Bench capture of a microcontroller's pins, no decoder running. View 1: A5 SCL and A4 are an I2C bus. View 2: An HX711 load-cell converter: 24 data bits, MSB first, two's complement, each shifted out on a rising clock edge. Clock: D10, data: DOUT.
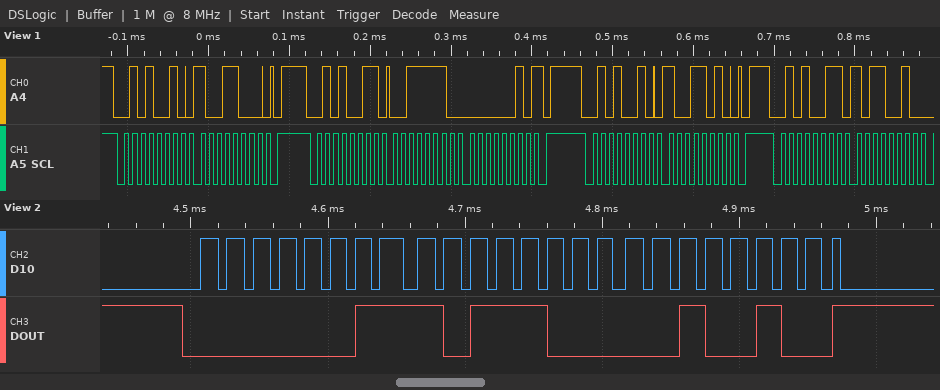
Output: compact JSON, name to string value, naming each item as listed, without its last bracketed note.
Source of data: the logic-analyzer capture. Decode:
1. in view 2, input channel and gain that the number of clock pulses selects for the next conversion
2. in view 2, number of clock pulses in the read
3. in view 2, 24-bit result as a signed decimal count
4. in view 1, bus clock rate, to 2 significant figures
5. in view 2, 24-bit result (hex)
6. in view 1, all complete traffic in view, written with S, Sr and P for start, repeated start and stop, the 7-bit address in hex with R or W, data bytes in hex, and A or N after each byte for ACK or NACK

{"in view 2, input channel and gain that the number of clock pulses selects for the next conversion": "channel A, gain 128", "in view 2, number of clock pulses in the read": "25", "in view 2, 24-bit result as a signed decimal count": "243748", "in view 1, bus clock rate, to 2 significant figures": "100 kHz", "in view 2, 24-bit result": "0x03B824", "in view 1, all complete traffic in view, written with S, Sr and P for start, repeated start and stop, the 7-bit address in hex with R or W, data bytes in hex, and A or N after each byte for ACK or NACK": "S 29W A 98 A P S 29R A 3E A 02 N P S 29W A 9A A P S 29R A B2 A"}
